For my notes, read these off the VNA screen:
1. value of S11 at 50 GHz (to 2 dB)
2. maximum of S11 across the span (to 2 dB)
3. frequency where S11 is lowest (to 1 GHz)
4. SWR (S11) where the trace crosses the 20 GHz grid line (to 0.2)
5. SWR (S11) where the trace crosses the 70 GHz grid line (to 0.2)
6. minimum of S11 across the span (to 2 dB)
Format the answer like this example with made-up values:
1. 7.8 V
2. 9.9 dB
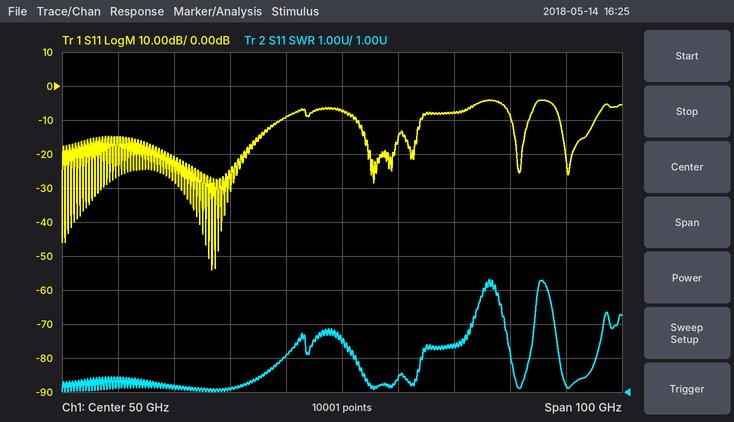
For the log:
1. -8 dB
2. -4 dB
3. 27 GHz
4. 1.2
5. 2.4
6. -54 dB
